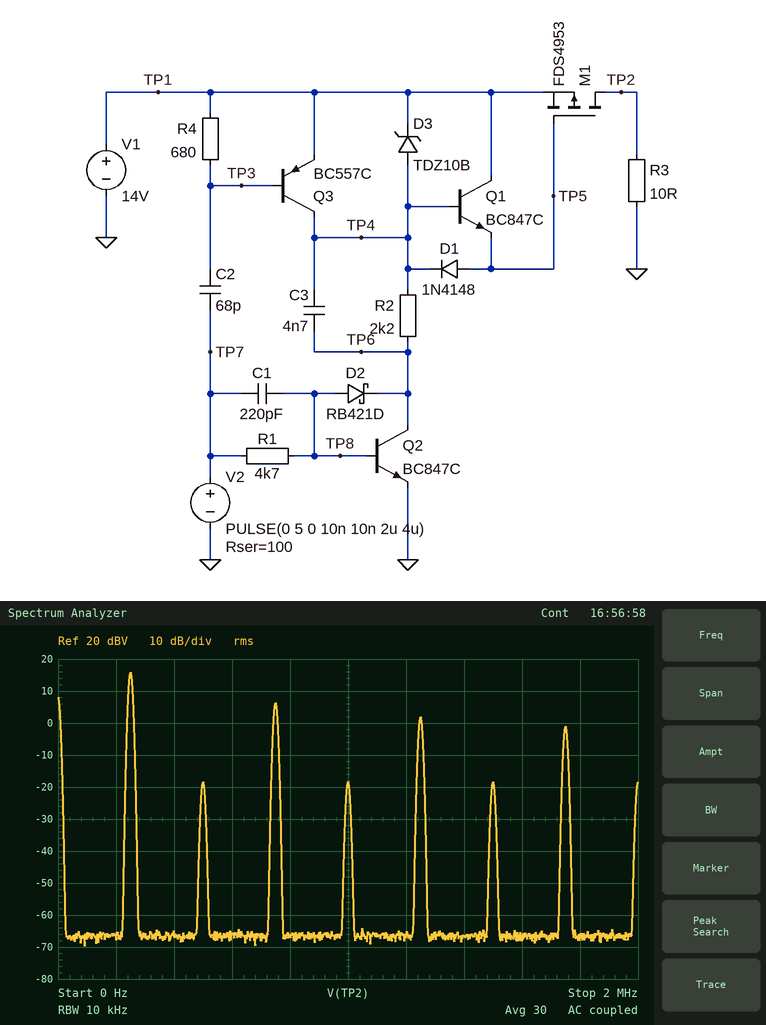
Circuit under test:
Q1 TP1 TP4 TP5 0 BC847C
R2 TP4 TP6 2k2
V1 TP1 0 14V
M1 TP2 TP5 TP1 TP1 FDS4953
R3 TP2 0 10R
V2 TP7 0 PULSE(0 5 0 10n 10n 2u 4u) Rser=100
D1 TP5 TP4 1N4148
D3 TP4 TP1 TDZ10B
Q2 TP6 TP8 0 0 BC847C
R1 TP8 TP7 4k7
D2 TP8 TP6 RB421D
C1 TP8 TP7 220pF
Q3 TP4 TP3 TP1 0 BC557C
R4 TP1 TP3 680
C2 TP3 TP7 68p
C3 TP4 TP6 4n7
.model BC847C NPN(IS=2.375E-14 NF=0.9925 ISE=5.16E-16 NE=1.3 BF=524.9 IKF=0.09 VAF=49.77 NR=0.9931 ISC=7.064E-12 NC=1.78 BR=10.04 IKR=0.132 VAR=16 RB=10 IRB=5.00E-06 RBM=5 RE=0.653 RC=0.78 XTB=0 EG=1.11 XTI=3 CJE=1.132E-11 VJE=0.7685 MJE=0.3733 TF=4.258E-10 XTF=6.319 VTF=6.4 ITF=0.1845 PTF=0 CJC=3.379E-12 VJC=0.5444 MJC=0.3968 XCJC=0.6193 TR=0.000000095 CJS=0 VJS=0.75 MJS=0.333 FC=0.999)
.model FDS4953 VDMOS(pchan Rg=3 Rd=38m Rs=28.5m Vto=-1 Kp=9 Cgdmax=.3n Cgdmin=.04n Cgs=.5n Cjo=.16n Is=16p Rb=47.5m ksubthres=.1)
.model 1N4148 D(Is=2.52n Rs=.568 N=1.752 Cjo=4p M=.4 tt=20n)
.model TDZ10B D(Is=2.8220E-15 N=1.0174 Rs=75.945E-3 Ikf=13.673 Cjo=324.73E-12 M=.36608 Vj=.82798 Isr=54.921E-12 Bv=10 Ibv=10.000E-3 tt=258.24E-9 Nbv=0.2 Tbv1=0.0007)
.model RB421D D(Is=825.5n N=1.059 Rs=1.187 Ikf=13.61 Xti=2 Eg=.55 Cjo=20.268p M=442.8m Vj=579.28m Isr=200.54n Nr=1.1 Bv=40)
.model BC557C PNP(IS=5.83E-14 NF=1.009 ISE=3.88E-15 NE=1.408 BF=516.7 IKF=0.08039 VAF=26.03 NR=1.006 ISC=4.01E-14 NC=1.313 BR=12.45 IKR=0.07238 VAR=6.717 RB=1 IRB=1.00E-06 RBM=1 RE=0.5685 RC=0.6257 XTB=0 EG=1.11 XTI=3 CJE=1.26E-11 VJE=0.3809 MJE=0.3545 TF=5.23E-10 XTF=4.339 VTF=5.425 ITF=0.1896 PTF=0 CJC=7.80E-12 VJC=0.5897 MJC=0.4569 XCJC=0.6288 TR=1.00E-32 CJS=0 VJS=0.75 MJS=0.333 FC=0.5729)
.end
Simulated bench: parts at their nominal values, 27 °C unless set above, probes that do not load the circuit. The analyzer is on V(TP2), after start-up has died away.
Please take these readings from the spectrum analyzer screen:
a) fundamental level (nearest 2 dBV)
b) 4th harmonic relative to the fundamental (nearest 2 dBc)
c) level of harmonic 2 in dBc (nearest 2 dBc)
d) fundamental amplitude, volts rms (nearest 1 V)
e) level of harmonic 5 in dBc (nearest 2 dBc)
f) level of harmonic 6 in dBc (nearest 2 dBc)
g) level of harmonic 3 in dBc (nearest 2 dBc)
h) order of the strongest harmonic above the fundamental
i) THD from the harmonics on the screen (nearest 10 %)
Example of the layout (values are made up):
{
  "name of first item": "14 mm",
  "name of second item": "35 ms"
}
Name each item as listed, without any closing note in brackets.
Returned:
{
  "fundamental level": "16 dBV",
  "4th harmonic relative to the fundamental": "-34 dBc",
  "level of harmonic 2 in dBc": "-34 dBc",
  "fundamental amplitude, volts rms": "6 V",
  "level of harmonic 5 in dBc": "-14 dBc",
  "level of harmonic 6 in dBc": "-34 dBc",
  "level of harmonic 3 in dBc": "-10 dBc",
  "order of the strongest harmonic above the fundamental": "3",
  "THD from the harmonics on the screen": "40 %"
}
